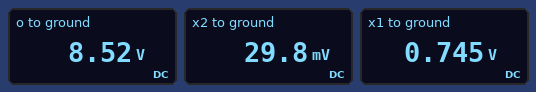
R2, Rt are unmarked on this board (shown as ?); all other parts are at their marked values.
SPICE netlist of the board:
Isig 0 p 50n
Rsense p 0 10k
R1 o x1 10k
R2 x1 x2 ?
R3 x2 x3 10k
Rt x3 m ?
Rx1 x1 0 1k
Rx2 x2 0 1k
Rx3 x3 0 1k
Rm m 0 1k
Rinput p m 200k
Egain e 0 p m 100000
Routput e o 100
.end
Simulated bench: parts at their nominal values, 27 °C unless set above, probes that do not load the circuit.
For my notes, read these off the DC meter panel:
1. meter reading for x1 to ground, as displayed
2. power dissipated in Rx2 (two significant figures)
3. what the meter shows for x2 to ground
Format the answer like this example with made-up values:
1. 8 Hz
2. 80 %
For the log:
1. 0.745 V
2. 890 nW
3. 29.8 mV
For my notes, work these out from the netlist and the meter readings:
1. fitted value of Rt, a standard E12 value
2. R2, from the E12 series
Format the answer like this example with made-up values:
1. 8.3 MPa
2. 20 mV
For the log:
1. 4.7 kΩ
2. 22 kΩ
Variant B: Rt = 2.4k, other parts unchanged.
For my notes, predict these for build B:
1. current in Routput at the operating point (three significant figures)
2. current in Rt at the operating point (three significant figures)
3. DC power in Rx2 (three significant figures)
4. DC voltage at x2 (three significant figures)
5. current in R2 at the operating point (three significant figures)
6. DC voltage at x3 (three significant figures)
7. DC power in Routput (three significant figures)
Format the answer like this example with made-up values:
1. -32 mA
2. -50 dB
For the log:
1. 541 µA
2. 437 nA
3. 429 nW
4. 20.7 mV
5. 22.6 µA
6. 1.49 mV
7. 29.3 µW
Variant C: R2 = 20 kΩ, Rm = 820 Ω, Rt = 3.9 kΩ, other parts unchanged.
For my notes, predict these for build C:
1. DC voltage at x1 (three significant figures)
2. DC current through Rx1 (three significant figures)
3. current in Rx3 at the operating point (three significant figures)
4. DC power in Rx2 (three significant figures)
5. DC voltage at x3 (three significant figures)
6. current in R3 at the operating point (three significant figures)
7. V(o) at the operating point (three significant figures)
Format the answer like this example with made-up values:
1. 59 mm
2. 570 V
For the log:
1. 713 mV
2. 713 µA
3. 2.38 µA
4. 973 nW
5. 2.38 mV
6. 2.88 µA
7. 8.18 V
